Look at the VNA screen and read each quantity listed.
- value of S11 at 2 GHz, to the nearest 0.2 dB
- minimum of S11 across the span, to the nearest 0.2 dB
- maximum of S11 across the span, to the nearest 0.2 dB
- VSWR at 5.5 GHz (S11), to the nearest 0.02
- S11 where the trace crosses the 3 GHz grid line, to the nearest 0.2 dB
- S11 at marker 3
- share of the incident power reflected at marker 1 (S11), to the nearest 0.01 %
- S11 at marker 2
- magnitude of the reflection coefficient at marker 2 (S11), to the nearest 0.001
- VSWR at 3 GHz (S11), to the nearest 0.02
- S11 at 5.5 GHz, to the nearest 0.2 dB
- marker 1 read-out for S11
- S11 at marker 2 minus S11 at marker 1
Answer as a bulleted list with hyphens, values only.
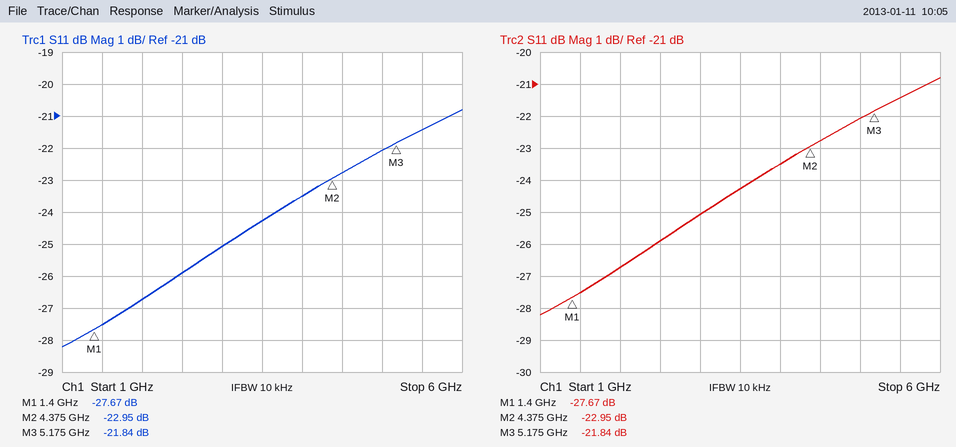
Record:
- -26.8 dB
- -28.2 dB
- -20.8 dB
- 1.18
- -25.0 dB
- -21.84 dB
- 0.17 %
- -22.95 dB
- 0.071
- 1.12
- -21.4 dB
- -27.67 dB
- 4.72 dB
